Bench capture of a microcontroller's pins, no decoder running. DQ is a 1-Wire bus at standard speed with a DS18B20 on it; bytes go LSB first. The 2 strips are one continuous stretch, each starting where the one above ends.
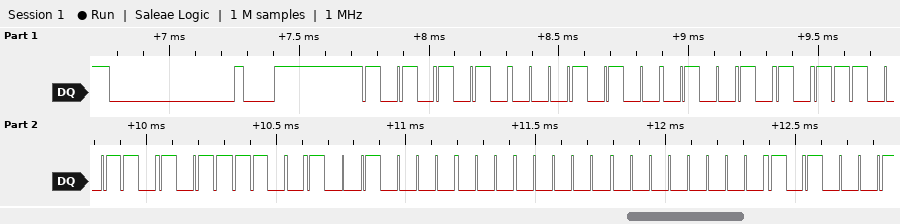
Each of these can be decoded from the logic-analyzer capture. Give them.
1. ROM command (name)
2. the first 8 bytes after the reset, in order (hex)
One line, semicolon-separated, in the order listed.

Match ROM; 55 28 52 67 3D 09 00 00
